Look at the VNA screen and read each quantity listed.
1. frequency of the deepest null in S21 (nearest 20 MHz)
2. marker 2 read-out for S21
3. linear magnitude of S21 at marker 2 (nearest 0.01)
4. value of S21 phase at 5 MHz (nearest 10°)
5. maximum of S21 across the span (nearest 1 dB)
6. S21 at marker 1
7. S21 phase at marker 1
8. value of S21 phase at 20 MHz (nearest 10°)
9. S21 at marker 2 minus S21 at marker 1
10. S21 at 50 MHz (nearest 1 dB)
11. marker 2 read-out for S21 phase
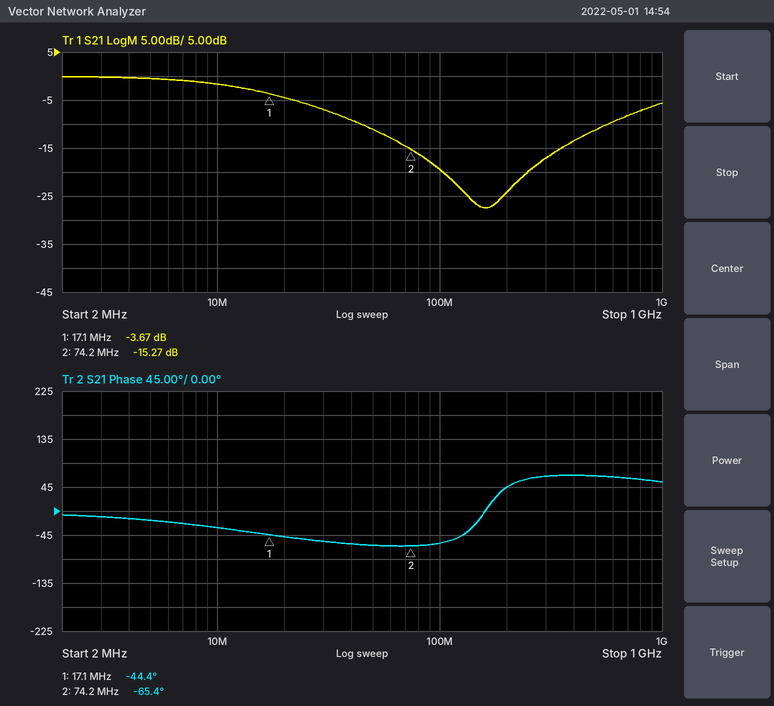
160 MHz
-15.27 dB
0.17
-20°
0 dB
-3.67 dB
-44.4°
-50°
-11.60 dB
-11 dB
-65.4°
